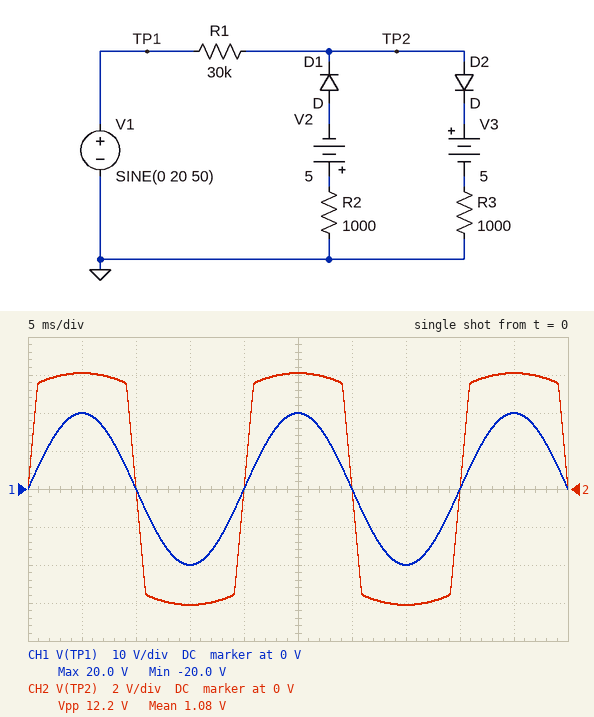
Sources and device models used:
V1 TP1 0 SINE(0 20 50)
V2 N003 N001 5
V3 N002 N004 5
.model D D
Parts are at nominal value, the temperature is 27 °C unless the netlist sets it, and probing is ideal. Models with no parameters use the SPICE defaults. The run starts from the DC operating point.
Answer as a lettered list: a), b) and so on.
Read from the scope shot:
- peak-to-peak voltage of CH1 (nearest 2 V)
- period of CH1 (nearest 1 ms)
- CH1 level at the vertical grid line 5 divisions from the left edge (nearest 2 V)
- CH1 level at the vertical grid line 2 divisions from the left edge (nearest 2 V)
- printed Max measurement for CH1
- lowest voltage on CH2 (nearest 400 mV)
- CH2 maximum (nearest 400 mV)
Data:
a) 40 V
b) 20 ms
c) 20 V
d) 0 V
e) 20.0 V
f) -6.0 V
g) 6.0 V
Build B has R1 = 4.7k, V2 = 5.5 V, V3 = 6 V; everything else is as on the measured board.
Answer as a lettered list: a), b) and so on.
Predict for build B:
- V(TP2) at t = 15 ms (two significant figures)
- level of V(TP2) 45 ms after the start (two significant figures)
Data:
a) -8.6 V
b) 9.0 V
